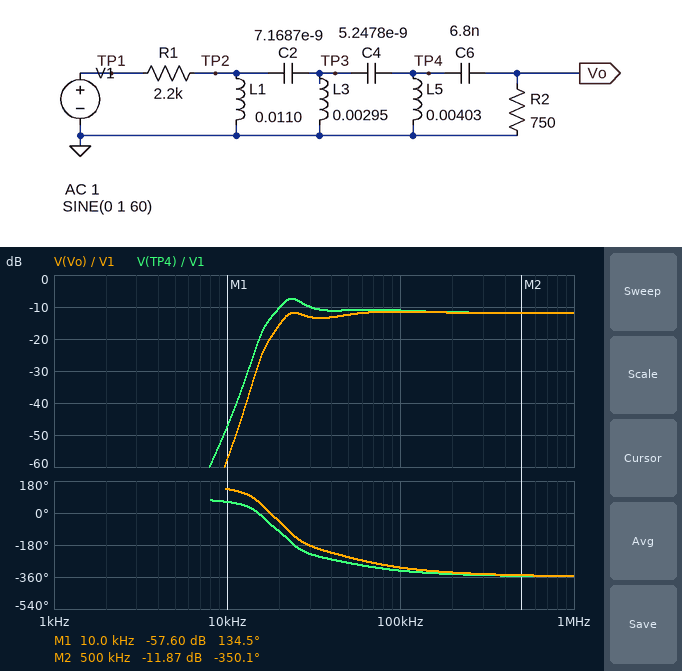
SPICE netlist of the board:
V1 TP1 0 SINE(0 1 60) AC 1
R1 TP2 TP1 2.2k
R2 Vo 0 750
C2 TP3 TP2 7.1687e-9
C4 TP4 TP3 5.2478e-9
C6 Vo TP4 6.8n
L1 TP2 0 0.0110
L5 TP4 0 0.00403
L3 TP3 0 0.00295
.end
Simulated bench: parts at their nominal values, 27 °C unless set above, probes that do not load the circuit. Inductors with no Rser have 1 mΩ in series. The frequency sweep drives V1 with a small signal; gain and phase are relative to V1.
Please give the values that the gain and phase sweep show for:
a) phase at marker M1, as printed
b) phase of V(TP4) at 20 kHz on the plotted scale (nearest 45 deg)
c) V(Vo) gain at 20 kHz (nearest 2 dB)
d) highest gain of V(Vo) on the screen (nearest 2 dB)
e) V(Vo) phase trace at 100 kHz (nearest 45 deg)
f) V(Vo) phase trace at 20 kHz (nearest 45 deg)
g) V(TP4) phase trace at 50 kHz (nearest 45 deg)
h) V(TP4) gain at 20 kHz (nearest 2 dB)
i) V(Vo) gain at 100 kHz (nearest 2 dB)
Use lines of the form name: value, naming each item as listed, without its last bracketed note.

phase at marker M1, as printed: 134.5 deg
phase of V(TP4) at 20 kHz on the plotted scale: -90 deg
V(Vo) gain at 20 kHz: -16 dB
highest gain of V(Vo) on the screen: -12 dB
V(Vo) phase trace at 100 kHz: -315 deg
V(Vo) phase trace at 20 kHz: -45 deg
V(TP4) phase trace at 50 kHz: -270 deg
V(TP4) gain at 20 kHz: -10 dB
V(Vo) gain at 100 kHz: -12 dB
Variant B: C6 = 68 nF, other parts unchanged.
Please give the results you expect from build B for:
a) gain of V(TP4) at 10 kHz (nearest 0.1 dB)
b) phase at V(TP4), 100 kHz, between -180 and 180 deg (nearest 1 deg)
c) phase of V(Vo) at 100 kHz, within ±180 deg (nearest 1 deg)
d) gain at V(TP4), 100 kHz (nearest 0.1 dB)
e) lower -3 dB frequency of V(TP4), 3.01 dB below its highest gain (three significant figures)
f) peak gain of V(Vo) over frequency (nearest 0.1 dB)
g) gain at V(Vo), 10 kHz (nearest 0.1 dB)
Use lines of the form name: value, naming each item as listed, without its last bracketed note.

gain of V(TP4) at 10 kHz: -47.9 dB
phase at V(TP4), 100 kHz, between -180 and 180 deg: 43 deg
phase of V(Vo) at 100 kHz, within ±180 deg: 44 deg
gain at V(TP4), 100 kHz: -12.1 dB
lower -3 dB frequency of V(TP4), 3.01 dB below its highest gain: 24.2 kHz
peak gain of V(Vo) over frequency: -11.6 dB
gain at V(Vo), 10 kHz: -48.3 dB
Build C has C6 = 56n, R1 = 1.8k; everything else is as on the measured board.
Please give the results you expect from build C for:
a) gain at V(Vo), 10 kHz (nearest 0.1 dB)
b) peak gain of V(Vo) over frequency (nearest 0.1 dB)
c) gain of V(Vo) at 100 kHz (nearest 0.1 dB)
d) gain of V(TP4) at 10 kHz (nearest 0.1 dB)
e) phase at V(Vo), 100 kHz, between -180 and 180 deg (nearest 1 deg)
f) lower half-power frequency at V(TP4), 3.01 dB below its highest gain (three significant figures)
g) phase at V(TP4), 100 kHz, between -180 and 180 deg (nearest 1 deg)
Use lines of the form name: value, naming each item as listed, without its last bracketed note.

gain at V(Vo), 10 kHz: -46.9 dB
peak gain of V(Vo) over frequency: -10.4 dB
gain of V(Vo) at 100 kHz: -10.8 dB
gain of V(TP4) at 10 kHz: -46.3 dB
phase at V(Vo), 100 kHz, between -180 and 180 deg: 45 deg
lower half-power frequency at V(TP4), 3.01 dB below its highest gain: 23.5 kHz
phase at V(TP4), 100 kHz, between -180 and 180 deg: 42 deg
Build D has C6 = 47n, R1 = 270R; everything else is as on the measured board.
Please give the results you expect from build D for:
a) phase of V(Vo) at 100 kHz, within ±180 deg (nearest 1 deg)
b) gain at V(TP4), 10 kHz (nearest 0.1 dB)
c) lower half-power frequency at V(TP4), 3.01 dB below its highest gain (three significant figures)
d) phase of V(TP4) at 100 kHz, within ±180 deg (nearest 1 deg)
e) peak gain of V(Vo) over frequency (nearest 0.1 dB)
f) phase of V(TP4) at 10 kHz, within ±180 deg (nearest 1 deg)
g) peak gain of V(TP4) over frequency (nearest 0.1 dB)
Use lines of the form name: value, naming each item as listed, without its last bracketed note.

phase of V(Vo) at 100 kHz, within ±180 deg: 45 deg
gain at V(TP4), 10 kHz: -40.5 dB
lower half-power frequency at V(TP4), 3.01 dB below its highest gain: 22.0 kHz
phase of V(TP4) at 100 kHz, within ±180 deg: 42 deg
peak gain of V(Vo) over frequency: -1.7 dB
phase of V(TP4) at 10 kHz, within ±180 deg: -5 deg
peak gain of V(TP4) over frequency: -1.6 dB
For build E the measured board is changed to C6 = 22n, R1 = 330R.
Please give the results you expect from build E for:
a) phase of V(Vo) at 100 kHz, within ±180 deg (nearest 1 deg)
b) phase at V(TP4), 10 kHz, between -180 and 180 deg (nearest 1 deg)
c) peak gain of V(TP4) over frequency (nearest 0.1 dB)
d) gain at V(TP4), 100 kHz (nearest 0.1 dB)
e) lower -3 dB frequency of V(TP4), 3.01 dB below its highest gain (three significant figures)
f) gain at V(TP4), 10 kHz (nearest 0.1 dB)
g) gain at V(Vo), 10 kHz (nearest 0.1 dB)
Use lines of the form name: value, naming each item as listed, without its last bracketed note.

phase of V(Vo) at 100 kHz, within ±180 deg: 46 deg
phase at V(TP4), 10 kHz, between -180 and 180 deg: 4 deg
peak gain of V(TP4) over frequency: -2.0 dB
gain at V(TP4), 100 kHz: -3.1 dB
lower -3 dB frequency of V(TP4), 3.01 dB below its highest gain: 21.4 kHz
gain at V(TP4), 10 kHz: -39.8 dB
gain at V(Vo), 10 kHz: -42.7 dB
